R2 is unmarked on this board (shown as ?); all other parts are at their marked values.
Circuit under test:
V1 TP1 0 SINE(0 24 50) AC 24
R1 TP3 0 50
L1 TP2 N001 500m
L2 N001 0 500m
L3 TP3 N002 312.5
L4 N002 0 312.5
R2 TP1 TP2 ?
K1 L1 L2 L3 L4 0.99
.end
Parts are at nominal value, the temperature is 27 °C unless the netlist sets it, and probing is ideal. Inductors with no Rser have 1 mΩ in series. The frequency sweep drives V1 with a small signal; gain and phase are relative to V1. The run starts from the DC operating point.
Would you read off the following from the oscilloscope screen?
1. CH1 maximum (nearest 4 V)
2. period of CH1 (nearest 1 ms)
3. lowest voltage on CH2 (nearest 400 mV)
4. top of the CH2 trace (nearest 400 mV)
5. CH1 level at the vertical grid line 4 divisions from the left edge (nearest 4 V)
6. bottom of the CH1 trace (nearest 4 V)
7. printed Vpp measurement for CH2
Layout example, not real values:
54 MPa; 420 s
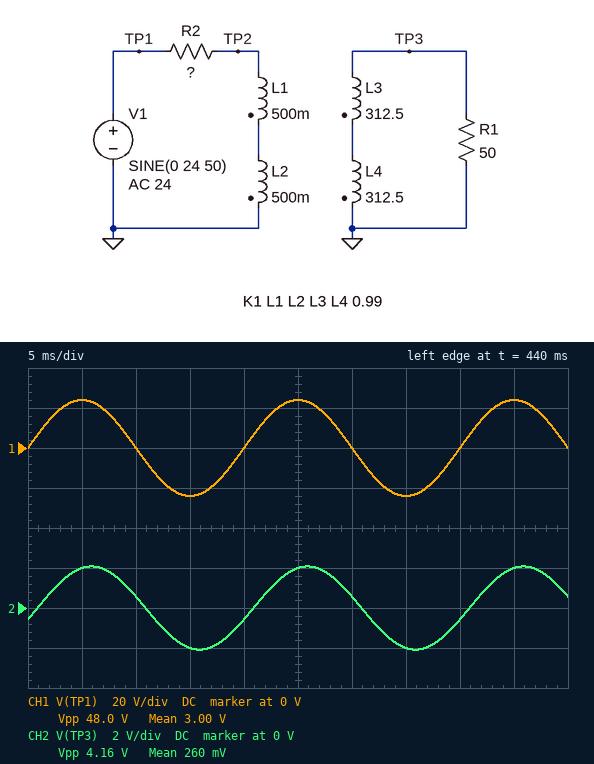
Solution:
24 V; 20 ms; -2.0 V; 2.0 V; 0 V; -24 V; 4.16 V
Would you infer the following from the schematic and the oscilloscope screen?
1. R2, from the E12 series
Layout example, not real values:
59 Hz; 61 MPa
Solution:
22 Ω
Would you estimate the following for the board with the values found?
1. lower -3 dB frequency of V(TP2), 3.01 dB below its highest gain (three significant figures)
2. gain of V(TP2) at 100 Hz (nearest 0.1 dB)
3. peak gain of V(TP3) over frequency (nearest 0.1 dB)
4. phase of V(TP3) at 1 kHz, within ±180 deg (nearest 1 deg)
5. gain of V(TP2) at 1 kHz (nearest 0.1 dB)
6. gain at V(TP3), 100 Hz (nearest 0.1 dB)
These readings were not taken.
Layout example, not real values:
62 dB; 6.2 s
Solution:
176 Hz; -6.1 dB; -20.9 dB; -80 deg; -0.1 dB; -22.1 dB
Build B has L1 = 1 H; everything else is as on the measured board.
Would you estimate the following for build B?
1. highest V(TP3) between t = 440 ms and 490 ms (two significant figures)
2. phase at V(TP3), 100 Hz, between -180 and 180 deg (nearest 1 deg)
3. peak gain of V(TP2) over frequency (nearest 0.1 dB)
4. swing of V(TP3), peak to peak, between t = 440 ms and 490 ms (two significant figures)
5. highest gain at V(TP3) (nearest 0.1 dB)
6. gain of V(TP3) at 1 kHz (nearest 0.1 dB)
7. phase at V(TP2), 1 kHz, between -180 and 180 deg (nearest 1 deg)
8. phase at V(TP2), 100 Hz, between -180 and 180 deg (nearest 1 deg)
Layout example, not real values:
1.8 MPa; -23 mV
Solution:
2.4 V; -40 deg; 0 dB; 4.8 V; -19.3 dB; -37.8 dB; 7 deg; 50 deg
